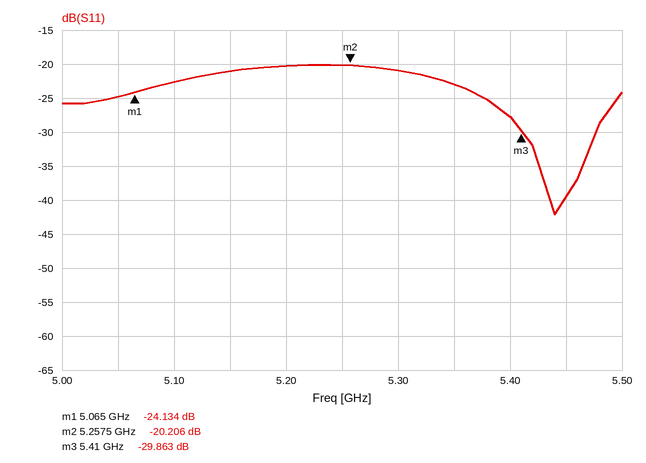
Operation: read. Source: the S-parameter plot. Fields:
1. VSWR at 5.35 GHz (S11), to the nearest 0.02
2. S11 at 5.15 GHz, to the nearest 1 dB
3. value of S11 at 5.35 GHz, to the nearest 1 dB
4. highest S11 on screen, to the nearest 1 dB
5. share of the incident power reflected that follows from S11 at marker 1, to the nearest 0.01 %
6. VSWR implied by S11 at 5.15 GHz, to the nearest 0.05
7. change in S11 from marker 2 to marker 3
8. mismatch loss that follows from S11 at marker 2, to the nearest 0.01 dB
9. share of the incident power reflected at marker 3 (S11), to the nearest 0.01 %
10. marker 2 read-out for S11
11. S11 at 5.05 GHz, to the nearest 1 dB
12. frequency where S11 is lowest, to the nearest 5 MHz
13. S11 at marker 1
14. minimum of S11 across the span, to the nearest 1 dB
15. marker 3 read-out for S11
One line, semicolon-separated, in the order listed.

1.16; -21 dB; -23 dB; -20 dB; 0.39 %; 1.20; -9.657 dB; 0.04 dB; 0.10 %; -20.206 dB; -25 dB; 5.440 GHz; -24.134 dB; -42 dB; -29.863 dB
